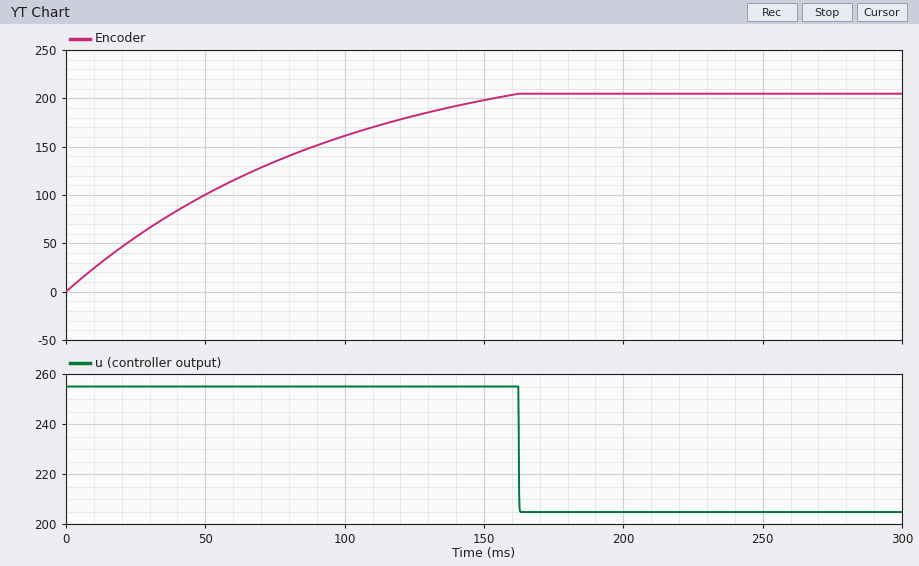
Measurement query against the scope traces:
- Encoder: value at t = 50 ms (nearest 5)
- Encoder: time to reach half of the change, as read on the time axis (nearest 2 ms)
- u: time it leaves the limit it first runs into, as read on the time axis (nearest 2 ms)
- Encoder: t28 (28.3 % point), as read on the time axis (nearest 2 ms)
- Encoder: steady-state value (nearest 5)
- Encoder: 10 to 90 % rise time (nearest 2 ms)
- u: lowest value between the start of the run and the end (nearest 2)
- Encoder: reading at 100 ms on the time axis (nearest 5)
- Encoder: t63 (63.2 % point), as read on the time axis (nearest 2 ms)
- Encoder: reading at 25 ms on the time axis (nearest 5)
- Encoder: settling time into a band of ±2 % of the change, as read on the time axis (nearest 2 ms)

100
52 ms
162 ms
26 ms
205
120 ms
204
160
70 ms
55
154 ms
